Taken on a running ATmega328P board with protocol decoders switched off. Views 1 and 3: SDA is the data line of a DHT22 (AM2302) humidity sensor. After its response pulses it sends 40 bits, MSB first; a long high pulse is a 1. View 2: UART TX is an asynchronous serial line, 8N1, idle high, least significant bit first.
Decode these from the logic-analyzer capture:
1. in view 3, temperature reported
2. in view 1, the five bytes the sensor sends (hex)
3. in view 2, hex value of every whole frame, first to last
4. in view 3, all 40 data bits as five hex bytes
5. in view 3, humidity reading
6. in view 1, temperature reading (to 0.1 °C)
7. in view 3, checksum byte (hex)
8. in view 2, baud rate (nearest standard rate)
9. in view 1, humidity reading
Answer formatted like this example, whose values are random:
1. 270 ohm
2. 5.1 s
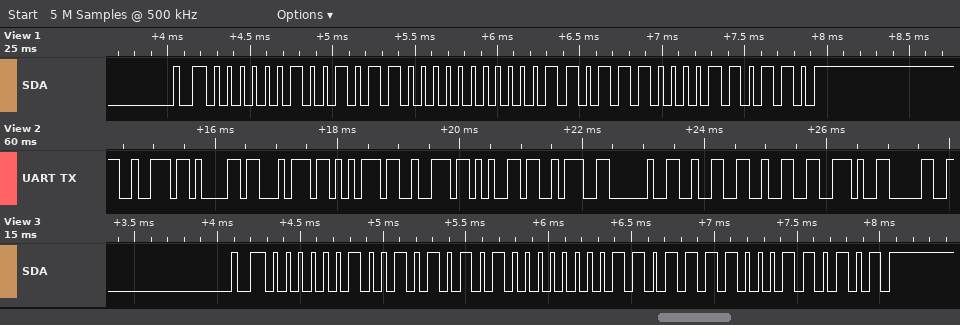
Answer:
1. 22.2 °C
2. 02 58 00 DC 36
3. 72 61 74 75 72 65 3A 20 32 32 2E 30
4. 02 55 00 DE 35
5. 59.7 %
6. 22.0 °C
7. 0x35
8. 9600 baud
9. 60.0 %
